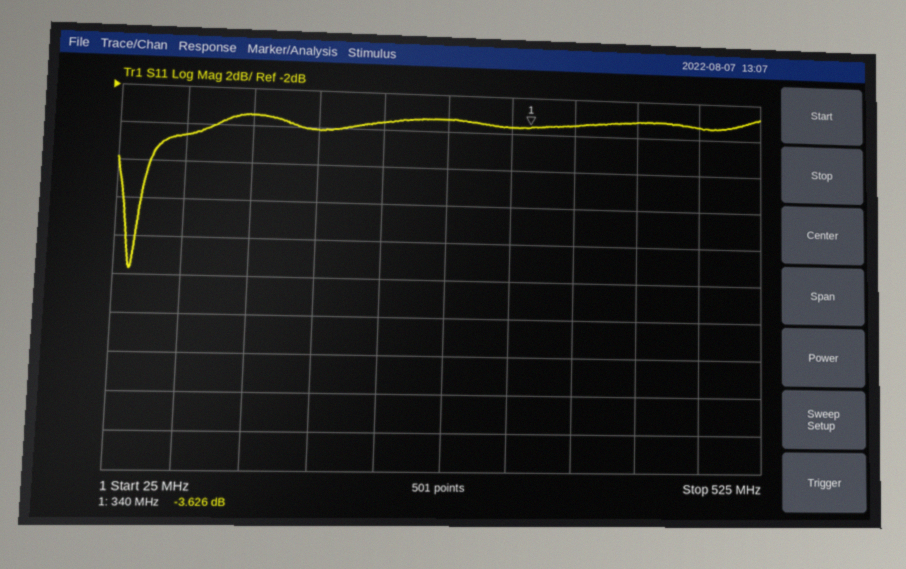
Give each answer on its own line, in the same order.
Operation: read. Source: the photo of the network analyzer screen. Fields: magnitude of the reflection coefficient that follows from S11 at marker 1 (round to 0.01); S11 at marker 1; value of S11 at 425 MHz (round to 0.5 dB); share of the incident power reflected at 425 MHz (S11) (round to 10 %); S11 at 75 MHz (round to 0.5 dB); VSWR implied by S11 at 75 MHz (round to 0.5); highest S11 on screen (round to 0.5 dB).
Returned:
0.66
-3.626 dB
-3.0 dB
50 %
-4.5 dB
4.0
-3.0 dB
